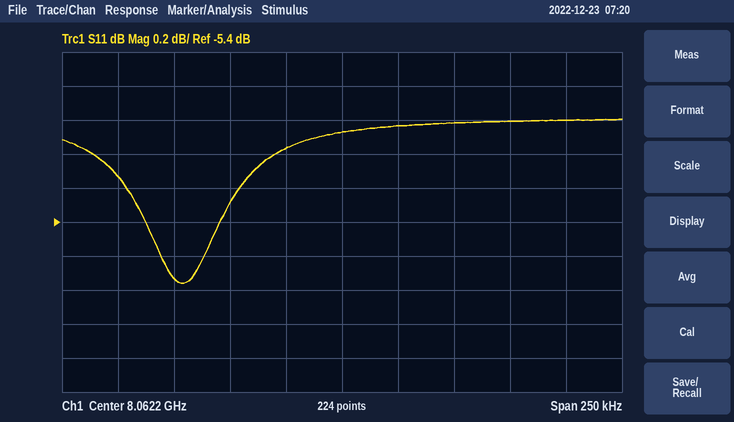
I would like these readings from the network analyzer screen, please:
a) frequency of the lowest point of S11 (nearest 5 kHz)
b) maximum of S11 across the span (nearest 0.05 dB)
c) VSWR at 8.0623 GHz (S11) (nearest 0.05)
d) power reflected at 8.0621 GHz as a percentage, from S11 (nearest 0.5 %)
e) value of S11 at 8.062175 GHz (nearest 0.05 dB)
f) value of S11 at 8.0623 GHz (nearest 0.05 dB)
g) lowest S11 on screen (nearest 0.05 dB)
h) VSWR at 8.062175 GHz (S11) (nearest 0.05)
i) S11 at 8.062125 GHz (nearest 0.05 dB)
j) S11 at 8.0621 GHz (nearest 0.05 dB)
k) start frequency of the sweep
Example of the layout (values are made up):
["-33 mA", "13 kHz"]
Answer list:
["8.062130 GHz", "-4.80 dB", "3.70", "30.5 %", "-4.95 dB", "-4.80 dB", "-5.75 dB", "3.60", "-5.75 dB", "-5.15 dB", "8.062075 GHz"]
